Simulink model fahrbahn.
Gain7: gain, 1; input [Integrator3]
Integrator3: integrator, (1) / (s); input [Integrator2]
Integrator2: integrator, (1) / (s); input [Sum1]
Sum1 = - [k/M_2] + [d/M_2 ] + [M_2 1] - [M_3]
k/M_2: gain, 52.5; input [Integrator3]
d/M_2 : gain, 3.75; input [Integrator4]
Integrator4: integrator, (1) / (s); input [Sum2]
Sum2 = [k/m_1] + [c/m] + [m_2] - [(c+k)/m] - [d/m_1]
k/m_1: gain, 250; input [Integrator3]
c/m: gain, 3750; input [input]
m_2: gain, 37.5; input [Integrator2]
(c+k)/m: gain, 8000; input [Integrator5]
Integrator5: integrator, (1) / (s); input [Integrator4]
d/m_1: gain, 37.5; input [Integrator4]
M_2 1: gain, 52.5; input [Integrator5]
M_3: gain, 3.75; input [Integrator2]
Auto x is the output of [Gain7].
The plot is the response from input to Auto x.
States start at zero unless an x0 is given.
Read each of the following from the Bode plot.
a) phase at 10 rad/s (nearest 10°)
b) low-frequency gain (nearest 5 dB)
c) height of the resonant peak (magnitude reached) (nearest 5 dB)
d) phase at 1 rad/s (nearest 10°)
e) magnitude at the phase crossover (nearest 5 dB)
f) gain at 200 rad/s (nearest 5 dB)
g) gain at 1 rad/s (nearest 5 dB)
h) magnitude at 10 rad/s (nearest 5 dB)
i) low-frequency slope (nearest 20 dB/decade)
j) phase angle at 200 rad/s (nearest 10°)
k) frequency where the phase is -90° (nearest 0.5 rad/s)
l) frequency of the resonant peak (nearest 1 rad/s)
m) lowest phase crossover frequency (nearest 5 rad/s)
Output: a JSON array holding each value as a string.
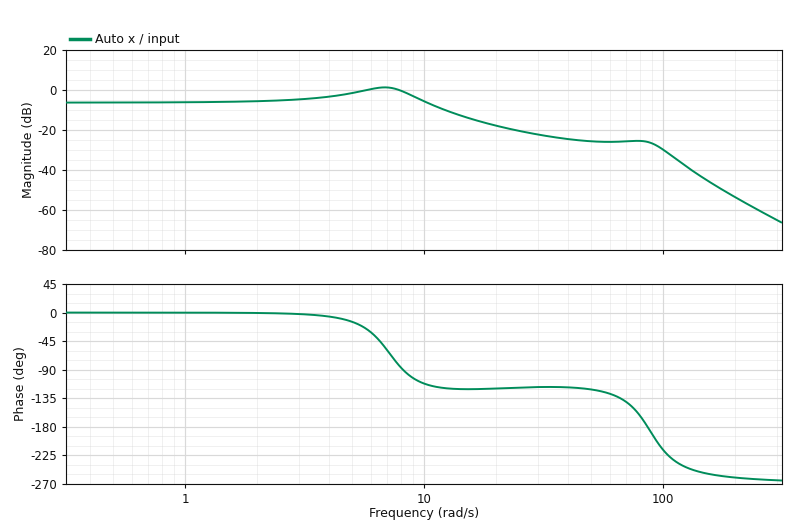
["-110°", "-5 dB", "0 dB", "0°", "-25 dB", "-55 dB", "-5 dB", "-5 dB", "0 dB/decade", "-260°", "8.0 rad/s", "7 rad/s", "85 rad/s"]
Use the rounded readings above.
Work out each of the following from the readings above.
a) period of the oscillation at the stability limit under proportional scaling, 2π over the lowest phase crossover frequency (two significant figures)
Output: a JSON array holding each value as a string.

["0.074 s"]
